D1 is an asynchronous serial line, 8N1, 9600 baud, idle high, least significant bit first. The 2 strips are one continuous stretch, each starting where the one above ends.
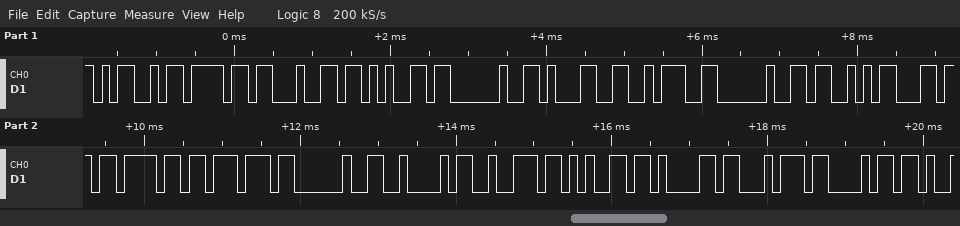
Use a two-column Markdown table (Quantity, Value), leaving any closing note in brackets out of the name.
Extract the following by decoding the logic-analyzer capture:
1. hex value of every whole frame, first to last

| Quantity | Value |
|---|---|
| hex value of every whole frame, first to last | 4D 6F 64 65 20 31 3A 20 53 6C 6F 77 20 42 72 65 61 74 68 |
